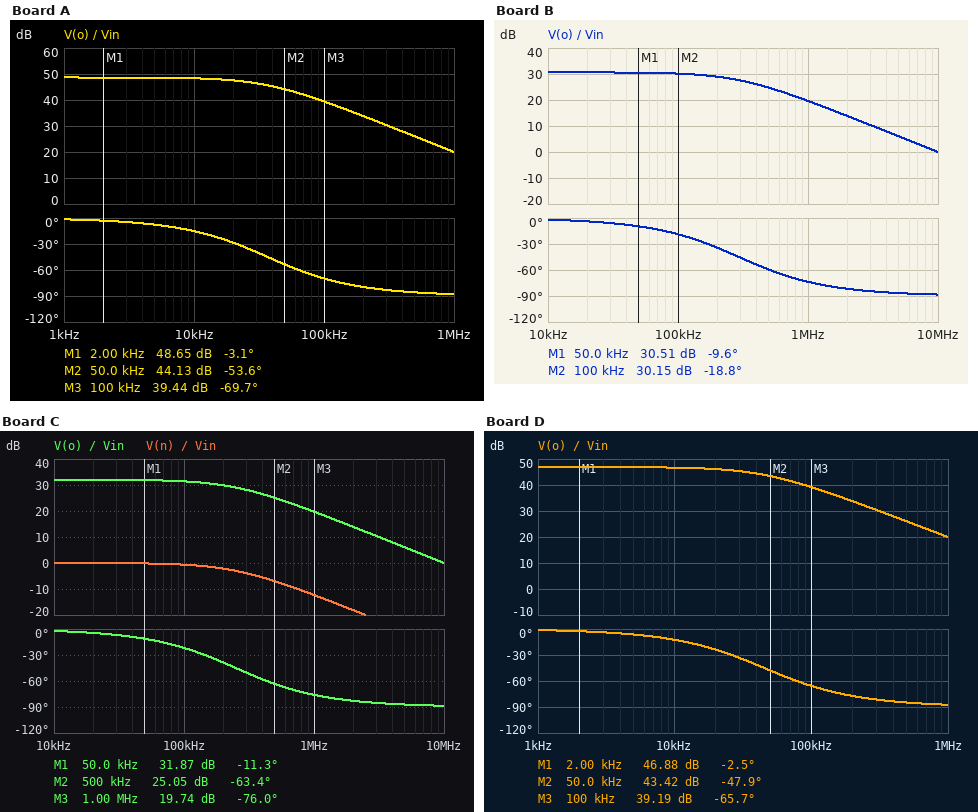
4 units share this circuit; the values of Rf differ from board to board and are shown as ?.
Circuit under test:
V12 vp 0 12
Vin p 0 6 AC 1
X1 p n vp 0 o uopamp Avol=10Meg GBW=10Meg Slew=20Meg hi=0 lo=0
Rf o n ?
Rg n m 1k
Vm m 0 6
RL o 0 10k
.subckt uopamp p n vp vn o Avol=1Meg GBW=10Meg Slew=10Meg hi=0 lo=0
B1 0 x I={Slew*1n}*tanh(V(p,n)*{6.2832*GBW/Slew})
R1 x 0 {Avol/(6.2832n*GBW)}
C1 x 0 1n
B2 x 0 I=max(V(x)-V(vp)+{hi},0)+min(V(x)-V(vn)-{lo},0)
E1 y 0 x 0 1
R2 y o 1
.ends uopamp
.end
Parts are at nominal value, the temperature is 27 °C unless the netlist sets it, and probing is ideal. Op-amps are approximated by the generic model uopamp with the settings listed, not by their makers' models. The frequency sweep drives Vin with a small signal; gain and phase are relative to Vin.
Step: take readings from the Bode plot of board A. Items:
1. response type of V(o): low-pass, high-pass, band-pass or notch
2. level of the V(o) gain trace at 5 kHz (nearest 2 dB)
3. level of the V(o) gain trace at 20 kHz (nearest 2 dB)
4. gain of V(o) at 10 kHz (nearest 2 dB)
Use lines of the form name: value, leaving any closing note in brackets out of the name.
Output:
response type of V(o): low-pass, high-pass, band-pass or notch: low-pass
level of the V(o) gain trace at 5 kHz: 48 dB
level of the V(o) gain trace at 20 kHz: 48 dB
gain of V(o) at 10 kHz: 48 dB
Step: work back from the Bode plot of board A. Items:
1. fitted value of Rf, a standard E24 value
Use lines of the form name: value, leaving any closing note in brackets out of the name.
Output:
fitted value of Rf, a standard E24 value: 270 kΩ
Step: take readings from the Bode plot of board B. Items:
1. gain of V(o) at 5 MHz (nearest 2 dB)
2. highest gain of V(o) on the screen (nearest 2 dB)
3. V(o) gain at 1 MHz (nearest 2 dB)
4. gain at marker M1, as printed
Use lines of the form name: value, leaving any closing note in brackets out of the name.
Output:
gain of V(o) at 5 MHz: 6 dB
highest gain of V(o) on the screen: 30 dB
V(o) gain at 1 MHz: 20 dB
gain at marker M1, as printed: 30.51 dB
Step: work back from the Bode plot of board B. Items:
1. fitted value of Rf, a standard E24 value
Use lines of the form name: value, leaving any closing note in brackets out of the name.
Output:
fitted value of Rf, a standard E24 value: 33 kΩ
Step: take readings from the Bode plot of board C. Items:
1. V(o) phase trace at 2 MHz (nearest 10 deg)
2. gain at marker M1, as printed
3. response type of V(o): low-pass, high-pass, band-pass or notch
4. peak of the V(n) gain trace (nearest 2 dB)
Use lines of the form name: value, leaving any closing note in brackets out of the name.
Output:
V(o) phase trace at 2 MHz: -80 deg
gain at marker M1, as printed: 31.87 dB
response type of V(o): low-pass, high-pass, band-pass or notch: low-pass
peak of the V(n) gain trace: 0 dB
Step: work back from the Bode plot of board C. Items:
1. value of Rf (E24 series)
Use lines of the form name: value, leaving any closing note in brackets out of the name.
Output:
value of Rf: 39 kΩ
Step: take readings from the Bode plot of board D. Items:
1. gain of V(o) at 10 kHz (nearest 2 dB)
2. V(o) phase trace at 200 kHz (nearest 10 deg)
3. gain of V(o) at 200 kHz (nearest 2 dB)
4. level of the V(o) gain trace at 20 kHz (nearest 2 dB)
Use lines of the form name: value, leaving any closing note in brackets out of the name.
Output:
gain of V(o) at 10 kHz: 46 dB
V(o) phase trace at 200 kHz: -80 deg
gain of V(o) at 200 kHz: 34 dB
level of the V(o) gain trace at 20 kHz: 46 dB
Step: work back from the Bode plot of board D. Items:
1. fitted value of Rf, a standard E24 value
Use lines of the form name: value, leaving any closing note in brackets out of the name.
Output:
fitted value of Rf, a standard E24 value: 220 kΩ
